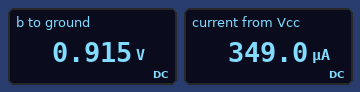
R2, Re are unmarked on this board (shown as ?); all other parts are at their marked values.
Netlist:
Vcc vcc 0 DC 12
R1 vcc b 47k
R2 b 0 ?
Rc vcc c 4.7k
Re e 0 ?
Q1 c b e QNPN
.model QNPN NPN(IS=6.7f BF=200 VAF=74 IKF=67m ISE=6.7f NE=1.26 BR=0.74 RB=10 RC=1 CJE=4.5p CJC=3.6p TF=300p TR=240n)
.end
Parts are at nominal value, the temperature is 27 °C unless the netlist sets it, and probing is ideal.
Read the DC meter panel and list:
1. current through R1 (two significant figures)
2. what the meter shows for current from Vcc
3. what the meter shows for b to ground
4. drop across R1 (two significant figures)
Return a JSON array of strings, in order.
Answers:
["240 µA", "349.0 µA", "0.915 V", "11 V"]
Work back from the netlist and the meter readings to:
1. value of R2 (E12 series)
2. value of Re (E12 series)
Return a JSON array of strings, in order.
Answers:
["3.9 kΩ", "2.7 kΩ"]
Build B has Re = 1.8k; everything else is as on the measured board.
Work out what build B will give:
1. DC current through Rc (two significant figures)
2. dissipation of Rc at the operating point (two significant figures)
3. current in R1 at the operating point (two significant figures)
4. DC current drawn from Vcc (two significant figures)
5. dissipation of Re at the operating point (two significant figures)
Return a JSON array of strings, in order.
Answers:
["160 µA", "130 µW", "240 µA", "400 µA", "49 µW"]
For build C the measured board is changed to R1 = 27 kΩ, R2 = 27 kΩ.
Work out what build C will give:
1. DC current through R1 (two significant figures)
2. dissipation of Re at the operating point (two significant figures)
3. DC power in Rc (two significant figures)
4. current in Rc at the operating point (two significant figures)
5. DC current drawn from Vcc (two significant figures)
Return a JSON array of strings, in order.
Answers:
["250 µA", "7.3 mW", "12 mW", "1.6 mA", "1.8 mA"]
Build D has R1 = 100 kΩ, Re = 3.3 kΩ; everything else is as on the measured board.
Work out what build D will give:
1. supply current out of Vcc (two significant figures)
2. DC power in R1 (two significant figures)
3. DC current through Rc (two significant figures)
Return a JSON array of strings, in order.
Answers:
["120 µA", "1.3 mW", "270 nA"]
